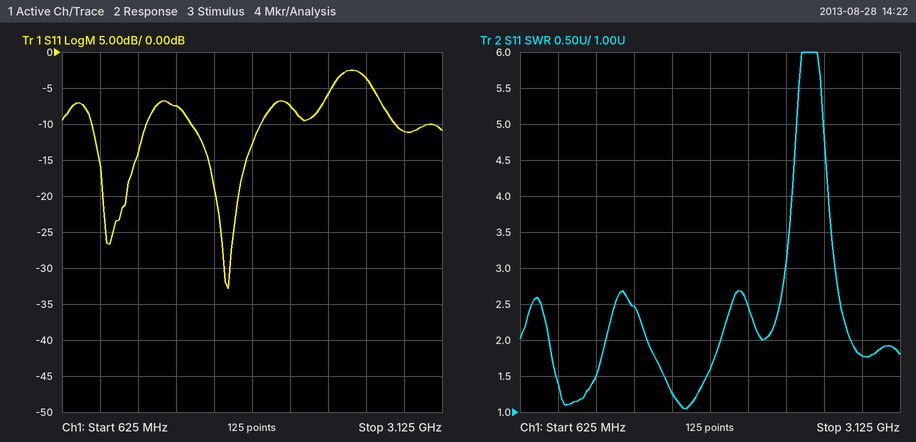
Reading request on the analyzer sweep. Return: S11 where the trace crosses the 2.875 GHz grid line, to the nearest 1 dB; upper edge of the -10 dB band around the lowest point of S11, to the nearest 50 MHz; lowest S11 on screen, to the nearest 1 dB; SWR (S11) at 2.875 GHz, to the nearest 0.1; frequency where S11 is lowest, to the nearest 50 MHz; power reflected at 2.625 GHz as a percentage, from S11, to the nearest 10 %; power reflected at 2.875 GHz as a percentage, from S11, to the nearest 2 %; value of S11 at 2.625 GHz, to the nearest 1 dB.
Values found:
-11 dB
1.95 GHz
-33 dB
1.8
1.70 GHz
40 %
8 %
-4 dB
